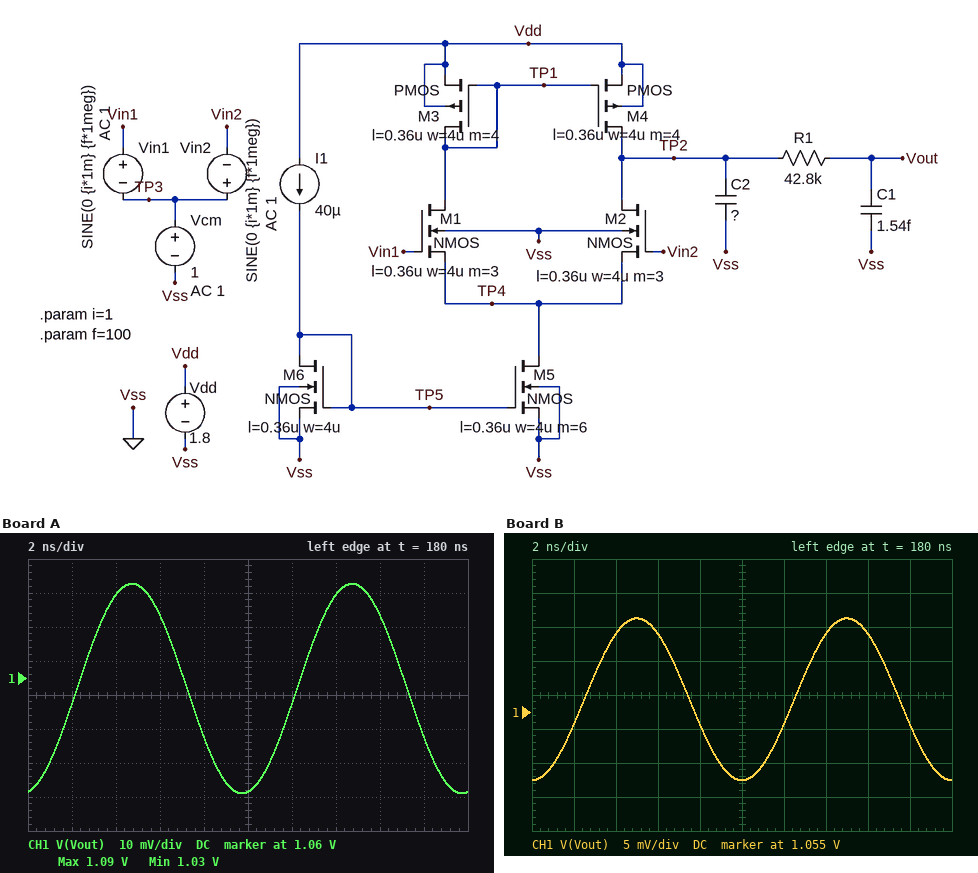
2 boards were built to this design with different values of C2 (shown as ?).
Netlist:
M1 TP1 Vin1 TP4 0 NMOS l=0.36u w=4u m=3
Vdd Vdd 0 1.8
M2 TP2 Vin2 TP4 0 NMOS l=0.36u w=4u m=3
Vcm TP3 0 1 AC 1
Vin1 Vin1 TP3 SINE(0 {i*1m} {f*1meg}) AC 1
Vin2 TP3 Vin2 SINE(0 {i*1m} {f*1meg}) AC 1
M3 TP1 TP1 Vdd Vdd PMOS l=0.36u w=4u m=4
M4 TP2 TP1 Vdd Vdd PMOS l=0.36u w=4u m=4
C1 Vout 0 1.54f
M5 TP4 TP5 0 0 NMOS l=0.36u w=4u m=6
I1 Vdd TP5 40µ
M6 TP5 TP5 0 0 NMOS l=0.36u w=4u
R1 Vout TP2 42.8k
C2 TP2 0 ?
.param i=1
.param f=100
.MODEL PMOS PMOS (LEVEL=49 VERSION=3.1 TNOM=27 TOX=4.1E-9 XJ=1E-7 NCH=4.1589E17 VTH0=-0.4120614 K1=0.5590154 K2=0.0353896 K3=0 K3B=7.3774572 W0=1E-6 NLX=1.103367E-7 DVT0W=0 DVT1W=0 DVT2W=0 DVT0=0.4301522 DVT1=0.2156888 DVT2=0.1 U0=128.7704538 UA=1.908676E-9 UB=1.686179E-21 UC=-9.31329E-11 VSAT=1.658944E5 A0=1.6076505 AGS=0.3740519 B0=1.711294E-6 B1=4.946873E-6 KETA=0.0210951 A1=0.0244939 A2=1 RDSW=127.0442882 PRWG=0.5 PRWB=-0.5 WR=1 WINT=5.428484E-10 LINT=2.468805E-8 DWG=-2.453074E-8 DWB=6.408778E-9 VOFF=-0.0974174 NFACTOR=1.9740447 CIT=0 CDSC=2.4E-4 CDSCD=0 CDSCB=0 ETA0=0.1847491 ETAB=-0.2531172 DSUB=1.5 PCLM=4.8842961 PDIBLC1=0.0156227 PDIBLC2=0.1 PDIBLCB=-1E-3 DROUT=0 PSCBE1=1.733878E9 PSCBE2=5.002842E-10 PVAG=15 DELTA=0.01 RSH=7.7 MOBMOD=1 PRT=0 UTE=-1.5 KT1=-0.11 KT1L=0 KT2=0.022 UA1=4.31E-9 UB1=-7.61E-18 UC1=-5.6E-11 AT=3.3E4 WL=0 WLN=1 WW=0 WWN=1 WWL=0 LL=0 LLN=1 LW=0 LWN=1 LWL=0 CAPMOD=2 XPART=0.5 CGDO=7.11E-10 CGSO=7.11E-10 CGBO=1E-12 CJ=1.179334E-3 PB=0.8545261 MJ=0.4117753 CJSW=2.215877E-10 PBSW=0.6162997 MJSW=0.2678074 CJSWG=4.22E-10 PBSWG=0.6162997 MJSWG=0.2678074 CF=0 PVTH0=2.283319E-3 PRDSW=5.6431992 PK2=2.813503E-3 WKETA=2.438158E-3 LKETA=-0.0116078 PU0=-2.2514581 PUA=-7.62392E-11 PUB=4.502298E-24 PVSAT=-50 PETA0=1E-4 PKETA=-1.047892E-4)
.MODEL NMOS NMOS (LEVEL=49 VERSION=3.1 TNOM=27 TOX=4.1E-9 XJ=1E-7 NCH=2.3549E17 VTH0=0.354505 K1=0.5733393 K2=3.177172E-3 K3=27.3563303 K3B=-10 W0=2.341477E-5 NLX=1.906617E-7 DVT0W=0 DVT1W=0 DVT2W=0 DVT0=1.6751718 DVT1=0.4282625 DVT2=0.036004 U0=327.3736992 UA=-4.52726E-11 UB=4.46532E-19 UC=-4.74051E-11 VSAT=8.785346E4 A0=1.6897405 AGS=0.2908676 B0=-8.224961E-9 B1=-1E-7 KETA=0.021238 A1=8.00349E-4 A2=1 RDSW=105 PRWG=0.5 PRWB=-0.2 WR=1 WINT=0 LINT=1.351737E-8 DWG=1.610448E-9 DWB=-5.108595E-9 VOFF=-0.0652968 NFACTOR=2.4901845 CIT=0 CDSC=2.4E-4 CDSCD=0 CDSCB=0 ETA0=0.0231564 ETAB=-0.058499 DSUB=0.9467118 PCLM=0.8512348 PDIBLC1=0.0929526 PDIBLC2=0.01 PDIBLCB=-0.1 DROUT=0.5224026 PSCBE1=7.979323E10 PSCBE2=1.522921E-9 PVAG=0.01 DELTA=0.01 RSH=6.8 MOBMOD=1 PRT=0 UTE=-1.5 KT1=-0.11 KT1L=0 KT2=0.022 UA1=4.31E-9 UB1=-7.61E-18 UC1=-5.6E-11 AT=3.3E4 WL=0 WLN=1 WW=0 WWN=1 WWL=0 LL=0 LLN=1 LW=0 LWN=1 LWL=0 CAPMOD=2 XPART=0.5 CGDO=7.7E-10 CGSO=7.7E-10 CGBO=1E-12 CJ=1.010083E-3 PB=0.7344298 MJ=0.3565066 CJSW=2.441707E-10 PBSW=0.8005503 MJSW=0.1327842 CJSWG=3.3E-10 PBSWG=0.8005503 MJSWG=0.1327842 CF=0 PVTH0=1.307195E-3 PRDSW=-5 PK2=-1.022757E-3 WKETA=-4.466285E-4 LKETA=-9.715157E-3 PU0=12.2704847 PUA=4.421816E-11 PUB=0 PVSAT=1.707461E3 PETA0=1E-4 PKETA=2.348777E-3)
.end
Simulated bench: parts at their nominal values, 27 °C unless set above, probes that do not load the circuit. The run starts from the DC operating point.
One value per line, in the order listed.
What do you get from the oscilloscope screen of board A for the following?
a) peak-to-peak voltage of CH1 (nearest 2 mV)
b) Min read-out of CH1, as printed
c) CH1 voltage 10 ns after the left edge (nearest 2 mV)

62 mV
1.03 V
1.026 V
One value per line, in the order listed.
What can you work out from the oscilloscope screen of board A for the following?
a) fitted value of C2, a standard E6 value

100 fF
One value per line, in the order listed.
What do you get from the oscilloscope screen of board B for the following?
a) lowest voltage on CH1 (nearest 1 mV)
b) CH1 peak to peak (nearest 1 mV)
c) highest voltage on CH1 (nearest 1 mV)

1.045 V
24 mV
1.069 V
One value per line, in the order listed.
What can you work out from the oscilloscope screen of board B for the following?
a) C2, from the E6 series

330 fF
